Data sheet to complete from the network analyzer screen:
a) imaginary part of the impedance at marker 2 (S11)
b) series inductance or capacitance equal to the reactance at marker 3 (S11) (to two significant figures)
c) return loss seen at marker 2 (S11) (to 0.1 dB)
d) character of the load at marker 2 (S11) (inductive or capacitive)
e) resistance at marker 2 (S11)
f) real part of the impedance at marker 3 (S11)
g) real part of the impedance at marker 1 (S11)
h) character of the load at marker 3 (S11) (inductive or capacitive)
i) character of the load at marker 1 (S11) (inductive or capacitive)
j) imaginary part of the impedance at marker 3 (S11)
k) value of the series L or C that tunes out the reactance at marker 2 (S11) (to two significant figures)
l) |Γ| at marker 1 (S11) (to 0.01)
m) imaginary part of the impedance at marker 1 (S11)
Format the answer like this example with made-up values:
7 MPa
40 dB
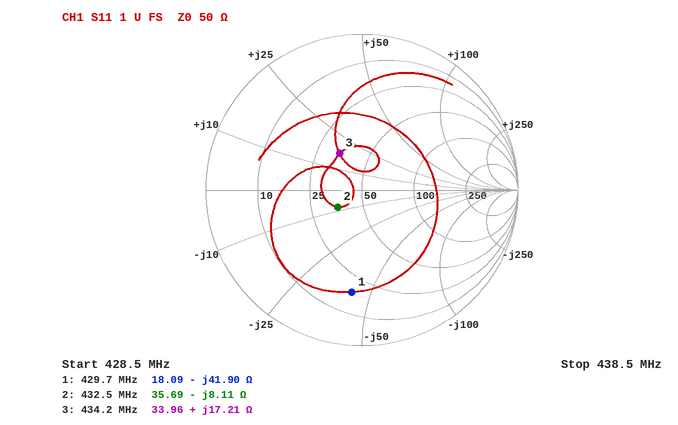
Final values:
-8.11 Ω
6.3 nH
14.4 dB
capacitive
35.69 Ω
33.96 Ω
18.09 Ω
inductive
capacitive
+17.21 Ω
3.0 nH
0.66
-41.90 Ω
